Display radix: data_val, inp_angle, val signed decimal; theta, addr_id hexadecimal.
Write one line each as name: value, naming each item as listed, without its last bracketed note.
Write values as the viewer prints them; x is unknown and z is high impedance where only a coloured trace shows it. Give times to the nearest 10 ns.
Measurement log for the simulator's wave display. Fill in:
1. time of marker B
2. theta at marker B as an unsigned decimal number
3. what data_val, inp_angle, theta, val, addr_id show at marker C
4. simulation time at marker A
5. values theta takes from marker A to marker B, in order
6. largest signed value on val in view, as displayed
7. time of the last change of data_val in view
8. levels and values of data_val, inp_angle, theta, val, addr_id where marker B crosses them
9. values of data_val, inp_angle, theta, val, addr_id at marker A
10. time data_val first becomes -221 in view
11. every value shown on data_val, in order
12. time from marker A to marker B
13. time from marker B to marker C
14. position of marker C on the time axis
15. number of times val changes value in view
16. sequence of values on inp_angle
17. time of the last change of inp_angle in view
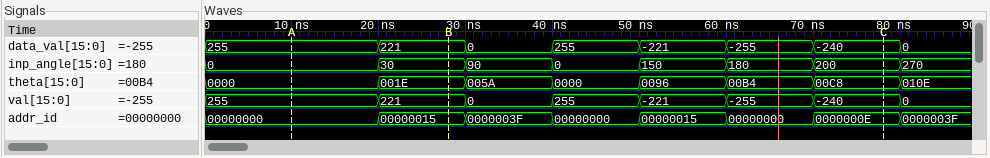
time of marker B: 30 ns
theta at marker B as an unsigned decimal number: 30
what data_val, inp_angle, theta, val, addr_id show at marker C: data_val=-240, inp_angle=200, theta=00C8, val=-240, addr_id=0000000E
simulation time at marker A: 10 ns
values theta takes from marker A to marker B, in order: 0000, 001E
largest signed value on val in view, as displayed: 255
time of the last change of data_val in view: 80 ns
levels and values of data_val, inp_angle, theta, val, addr_id where marker B crosses them: data_val=221, inp_angle=30, theta=001E, val=221, addr_id=00000015
values of data_val, inp_angle, theta, val, addr_id at marker A: data_val=255, inp_angle=0, theta=0000, val=255, addr_id=00000000
time data_val first becomes -221 in view: 50 ns
every value shown on data_val, in order: 255, 221, 0, 255, -221, -255, -240, 0
time from marker A to marker B: 20 ns
time from marker B to marker C: 50 ns
position of marker C on the time axis: 80 ns
number of times val changes value in view: 7
sequence of values on inp_angle: 0, 30, 90, 0, 150, 180, 200, 270
time of the last change of inp_angle in view: 80 ns
